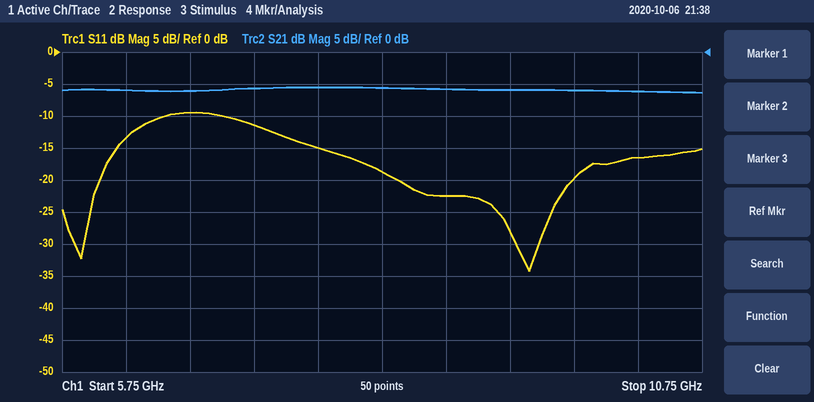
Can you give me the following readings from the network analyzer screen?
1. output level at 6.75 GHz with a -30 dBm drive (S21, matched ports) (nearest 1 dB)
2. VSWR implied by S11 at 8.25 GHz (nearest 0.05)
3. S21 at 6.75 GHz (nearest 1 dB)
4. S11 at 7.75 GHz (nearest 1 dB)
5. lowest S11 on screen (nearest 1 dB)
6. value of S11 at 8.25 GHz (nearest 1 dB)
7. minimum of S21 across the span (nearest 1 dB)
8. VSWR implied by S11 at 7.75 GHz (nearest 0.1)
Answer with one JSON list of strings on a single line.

["-36 dBm", "1.25", "-6 dB", "-15 dB", "-34 dB", "-19 dB", "-6 dB", "1.4"]
